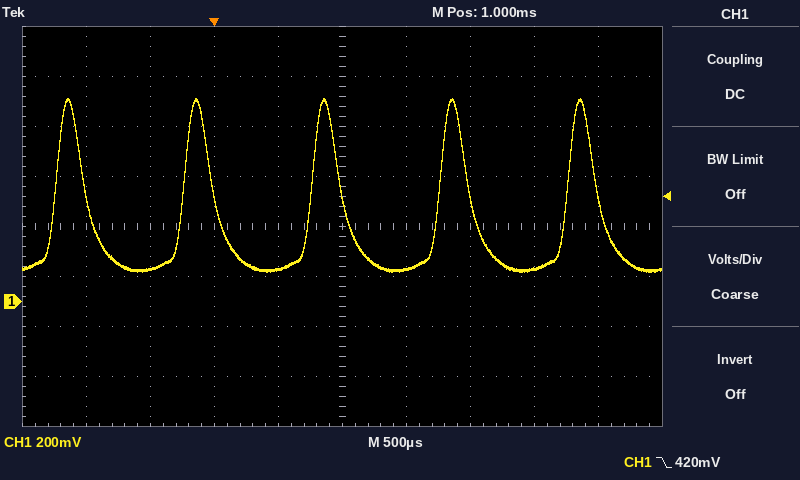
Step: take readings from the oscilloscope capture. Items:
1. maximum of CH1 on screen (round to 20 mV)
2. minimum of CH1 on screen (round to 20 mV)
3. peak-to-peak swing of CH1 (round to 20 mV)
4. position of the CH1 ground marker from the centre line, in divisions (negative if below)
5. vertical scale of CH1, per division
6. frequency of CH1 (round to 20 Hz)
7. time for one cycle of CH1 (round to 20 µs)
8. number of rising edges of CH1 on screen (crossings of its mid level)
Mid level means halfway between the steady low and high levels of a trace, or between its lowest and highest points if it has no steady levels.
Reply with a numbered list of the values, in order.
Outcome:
1. 820 mV
2. 120 mV
3. 700 mV
4. -1.5 div
5. 200 mV
6. 1.00 kHz
7. 1.00 ms
8. 5
